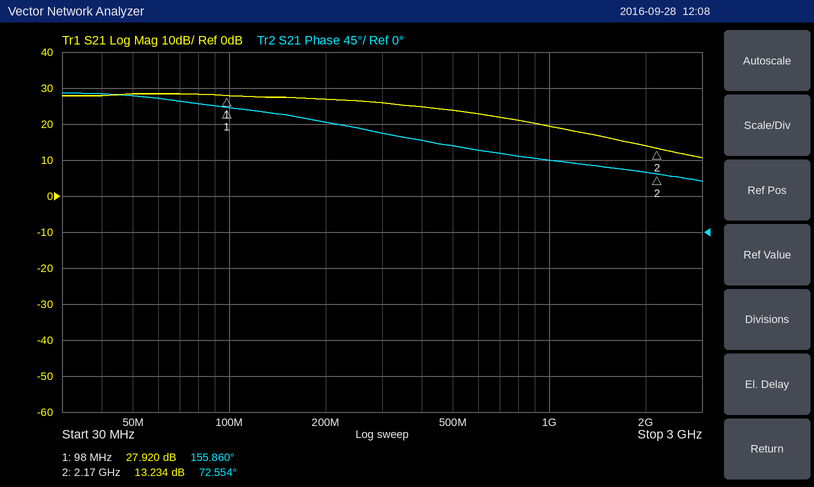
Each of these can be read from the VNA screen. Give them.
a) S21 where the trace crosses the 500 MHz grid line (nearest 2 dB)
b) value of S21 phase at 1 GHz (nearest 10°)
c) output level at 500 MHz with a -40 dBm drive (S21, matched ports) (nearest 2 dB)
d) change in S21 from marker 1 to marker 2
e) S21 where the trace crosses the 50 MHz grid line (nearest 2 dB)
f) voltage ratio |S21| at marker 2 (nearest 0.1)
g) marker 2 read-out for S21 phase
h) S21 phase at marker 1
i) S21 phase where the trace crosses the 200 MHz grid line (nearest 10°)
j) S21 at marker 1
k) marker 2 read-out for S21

24 dB
90°
-16 dBm
-14.686 dB
28 dB
4.6
72.554°
155.860°
140°
27.920 dB
13.234 dB
